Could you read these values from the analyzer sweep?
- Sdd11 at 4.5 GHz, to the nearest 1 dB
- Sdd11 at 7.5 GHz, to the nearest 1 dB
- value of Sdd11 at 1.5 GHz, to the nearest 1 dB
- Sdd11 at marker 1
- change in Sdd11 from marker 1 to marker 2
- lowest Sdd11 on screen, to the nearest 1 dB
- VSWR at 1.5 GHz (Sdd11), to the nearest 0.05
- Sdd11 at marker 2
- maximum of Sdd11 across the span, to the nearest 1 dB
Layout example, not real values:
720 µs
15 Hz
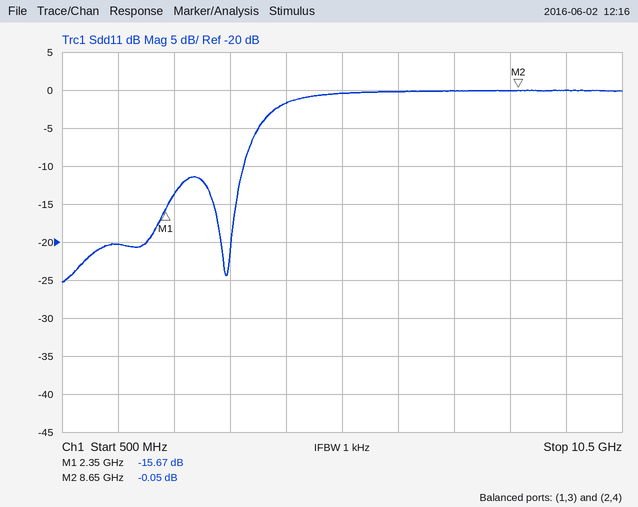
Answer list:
-2 dB
0 dB
-20 dB
-15.67 dB
15.62 dB
-25 dB
1.20
-0.05 dB
0 dB
